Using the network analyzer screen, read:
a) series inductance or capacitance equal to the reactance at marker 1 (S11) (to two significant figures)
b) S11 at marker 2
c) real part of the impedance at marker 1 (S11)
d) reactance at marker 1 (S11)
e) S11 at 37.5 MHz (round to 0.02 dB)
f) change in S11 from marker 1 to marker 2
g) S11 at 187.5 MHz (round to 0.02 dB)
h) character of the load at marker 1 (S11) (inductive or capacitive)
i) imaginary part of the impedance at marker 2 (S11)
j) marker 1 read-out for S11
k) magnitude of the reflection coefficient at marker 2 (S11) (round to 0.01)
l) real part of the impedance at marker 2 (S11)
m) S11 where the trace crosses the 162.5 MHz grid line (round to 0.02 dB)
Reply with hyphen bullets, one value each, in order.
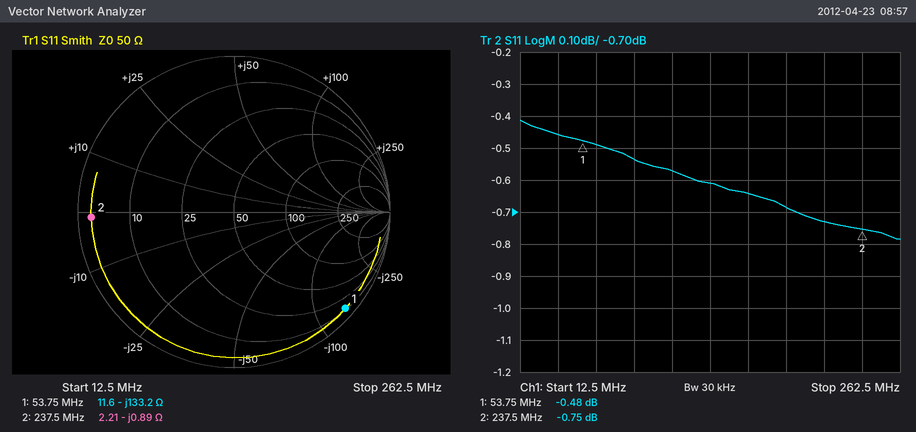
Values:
- 22 pF
- -0.75 dB
- 11.6 Ω
- -133.2 Ω
- -0.46 dB
- -0.27 dB
- -0.68 dB
- capacitive
- -0.89 Ω
- -0.48 dB
- 0.92
- 2.21 Ω
- -0.64 dB
